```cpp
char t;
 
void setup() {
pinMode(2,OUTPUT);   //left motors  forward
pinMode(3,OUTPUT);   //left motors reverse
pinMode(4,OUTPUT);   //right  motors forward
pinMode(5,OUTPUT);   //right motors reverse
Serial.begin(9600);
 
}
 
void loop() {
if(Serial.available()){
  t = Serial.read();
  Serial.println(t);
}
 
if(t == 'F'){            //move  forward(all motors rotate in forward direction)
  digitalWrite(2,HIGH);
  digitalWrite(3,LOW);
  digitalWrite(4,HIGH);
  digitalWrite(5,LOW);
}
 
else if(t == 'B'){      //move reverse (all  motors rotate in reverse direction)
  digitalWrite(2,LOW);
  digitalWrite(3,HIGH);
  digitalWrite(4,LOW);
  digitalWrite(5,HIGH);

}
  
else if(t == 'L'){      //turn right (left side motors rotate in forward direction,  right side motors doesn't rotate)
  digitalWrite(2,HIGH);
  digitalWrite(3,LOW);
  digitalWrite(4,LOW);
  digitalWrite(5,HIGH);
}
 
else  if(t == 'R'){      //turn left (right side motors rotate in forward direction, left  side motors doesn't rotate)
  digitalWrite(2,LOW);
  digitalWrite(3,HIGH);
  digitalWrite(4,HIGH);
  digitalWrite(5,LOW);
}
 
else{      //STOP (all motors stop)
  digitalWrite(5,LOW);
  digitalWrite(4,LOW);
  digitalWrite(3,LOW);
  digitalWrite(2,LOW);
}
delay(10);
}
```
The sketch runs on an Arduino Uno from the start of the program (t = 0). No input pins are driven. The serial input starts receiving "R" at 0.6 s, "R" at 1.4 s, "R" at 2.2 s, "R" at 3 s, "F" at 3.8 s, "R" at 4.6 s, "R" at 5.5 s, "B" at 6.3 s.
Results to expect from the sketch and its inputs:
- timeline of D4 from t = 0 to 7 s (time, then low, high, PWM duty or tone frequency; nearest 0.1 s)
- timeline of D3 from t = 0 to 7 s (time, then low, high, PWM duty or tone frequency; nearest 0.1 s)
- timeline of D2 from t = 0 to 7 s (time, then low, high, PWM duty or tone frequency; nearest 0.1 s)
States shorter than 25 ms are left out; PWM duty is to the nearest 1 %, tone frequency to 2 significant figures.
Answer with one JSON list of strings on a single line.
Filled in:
["0 s low; 0.6 s high; 6.3 s low", "0 s low; 0.6 s high; 3.8 s low; 4.6 s high", "0 s low; 3.8 s high; 4.6 s low"]
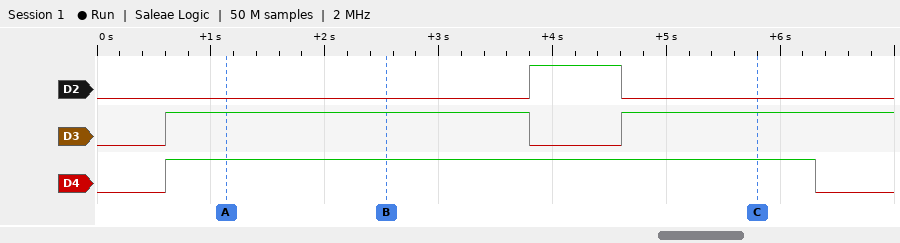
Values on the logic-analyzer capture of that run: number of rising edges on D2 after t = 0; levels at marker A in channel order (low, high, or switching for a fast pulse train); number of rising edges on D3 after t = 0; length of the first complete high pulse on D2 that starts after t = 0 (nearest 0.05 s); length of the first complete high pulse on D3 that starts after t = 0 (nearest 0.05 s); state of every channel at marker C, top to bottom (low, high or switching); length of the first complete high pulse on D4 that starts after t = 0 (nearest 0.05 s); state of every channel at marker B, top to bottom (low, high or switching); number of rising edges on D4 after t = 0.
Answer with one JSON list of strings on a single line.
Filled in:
["1", "D2 low, D3 high, D4 high", "2", "0.80 s", "3.20 s", "D2 low, D3 high, D4 high", "5.70 s", "D2 low, D3 high, D4 high", "1"]
